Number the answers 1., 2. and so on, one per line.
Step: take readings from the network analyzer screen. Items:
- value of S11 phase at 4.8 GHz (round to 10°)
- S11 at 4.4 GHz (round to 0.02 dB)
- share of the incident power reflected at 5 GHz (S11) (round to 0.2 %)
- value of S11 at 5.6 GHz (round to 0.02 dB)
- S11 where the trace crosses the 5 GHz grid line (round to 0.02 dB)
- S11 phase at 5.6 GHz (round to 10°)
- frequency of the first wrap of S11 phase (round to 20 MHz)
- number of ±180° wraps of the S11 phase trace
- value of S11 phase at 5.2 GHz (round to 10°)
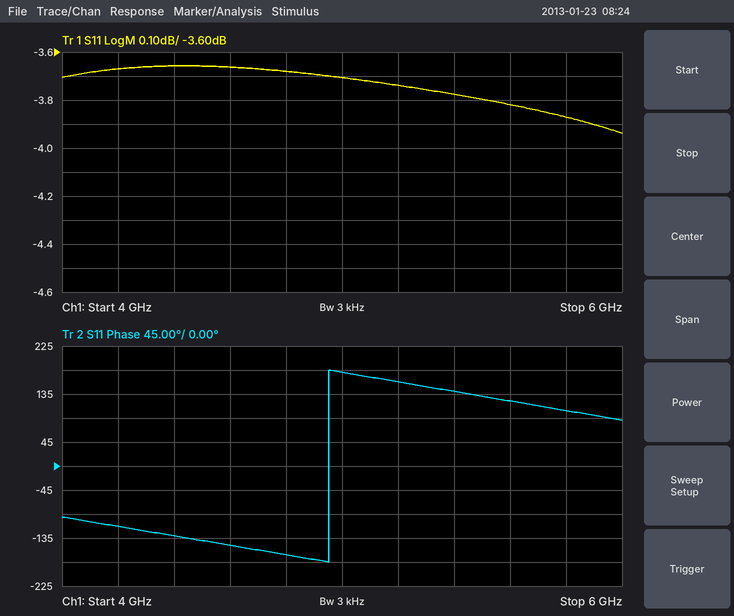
1. -170°
2. -3.66 dB
3. 42.6 %
4. -3.82 dB
5. -3.70 dB
6. 120°
7. 4.96 GHz
8. 1
9. 160°
